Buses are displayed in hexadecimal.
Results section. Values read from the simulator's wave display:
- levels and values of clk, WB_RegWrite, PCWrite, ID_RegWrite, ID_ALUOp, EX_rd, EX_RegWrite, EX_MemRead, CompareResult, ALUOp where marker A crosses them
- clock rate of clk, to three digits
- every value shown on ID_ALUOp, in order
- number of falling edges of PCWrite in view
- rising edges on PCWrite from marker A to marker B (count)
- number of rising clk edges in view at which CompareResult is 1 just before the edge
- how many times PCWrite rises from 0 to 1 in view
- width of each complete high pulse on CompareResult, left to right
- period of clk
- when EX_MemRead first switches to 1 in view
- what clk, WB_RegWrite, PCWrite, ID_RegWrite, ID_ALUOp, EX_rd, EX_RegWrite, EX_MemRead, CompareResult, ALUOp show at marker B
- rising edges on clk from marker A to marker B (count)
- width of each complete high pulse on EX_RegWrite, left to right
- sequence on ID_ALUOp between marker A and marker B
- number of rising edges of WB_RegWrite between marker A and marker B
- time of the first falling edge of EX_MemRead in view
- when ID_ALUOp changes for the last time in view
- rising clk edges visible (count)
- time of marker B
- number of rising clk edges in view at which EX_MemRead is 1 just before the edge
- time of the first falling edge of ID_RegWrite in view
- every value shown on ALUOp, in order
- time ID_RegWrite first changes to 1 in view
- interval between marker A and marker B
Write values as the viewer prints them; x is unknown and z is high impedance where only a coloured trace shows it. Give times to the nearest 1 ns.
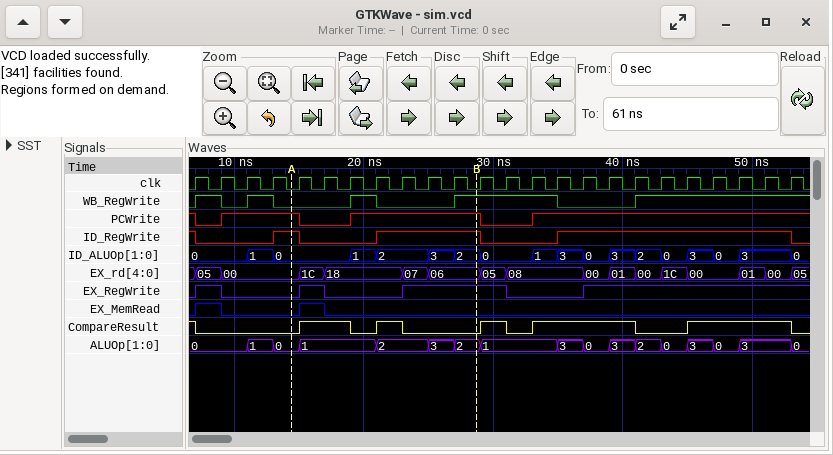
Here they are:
clk=0, WB_RegWrite=0, PCWrite=1, ID_RegWrite=1, ID_ALUOp=0, EX_rd=00, EX_RegWrite=0, EX_MemRead=0, CompareResult=0, ALUOp=0
500 MHz
0, 1, 0, 1, 2, 3, 2, 0, 1, 3, 0, 3, 2, 0, 3, 0, 3, 0
3
1
13
3
4 ns, 2 ns, 2 ns, 8 ns, 8 ns
2 ns
7 ns
clk=0, WB_RegWrite=1, PCWrite=1, ID_RegWrite=1, ID_ALUOp=2, EX_rd=06, EX_RegWrite=1, EX_MemRead=0, CompareResult=0, ALUOp=2
7
2 ns, 2 ns, 8 ns
0, 1, 2, 3, 2
2
9 ns
53 ns
24
29 ns
2
7 ns
0, 1, 0, 1, 2, 3, 2, 1, 3, 0, 3, 2, 0, 3, 0, 3, 0
13 ns
14 ns
